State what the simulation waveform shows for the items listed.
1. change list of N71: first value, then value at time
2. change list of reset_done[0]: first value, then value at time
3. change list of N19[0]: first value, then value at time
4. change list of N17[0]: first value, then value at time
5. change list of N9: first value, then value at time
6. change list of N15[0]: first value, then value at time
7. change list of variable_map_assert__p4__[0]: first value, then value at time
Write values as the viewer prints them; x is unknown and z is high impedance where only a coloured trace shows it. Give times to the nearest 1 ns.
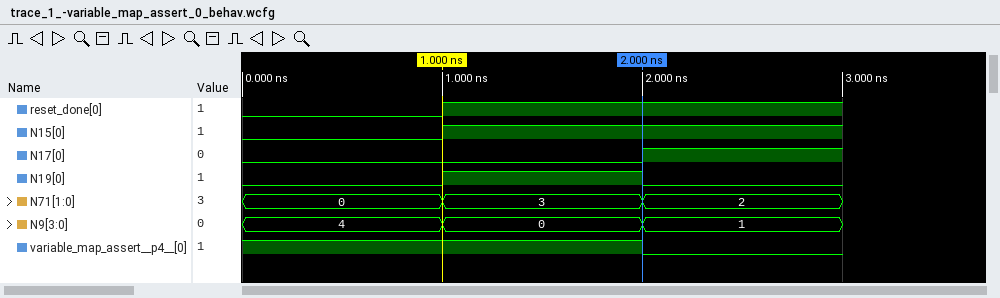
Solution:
0, 3 at 1 ns, 2 at 2 ns
0, 1 at 1 ns
0, 1 at 1 ns, 0 at 2 ns
0, 1 at 2 ns
4, 0 at 1 ns, 1 at 2 ns
0, 1 at 1 ns
1, 0 at 2 ns
